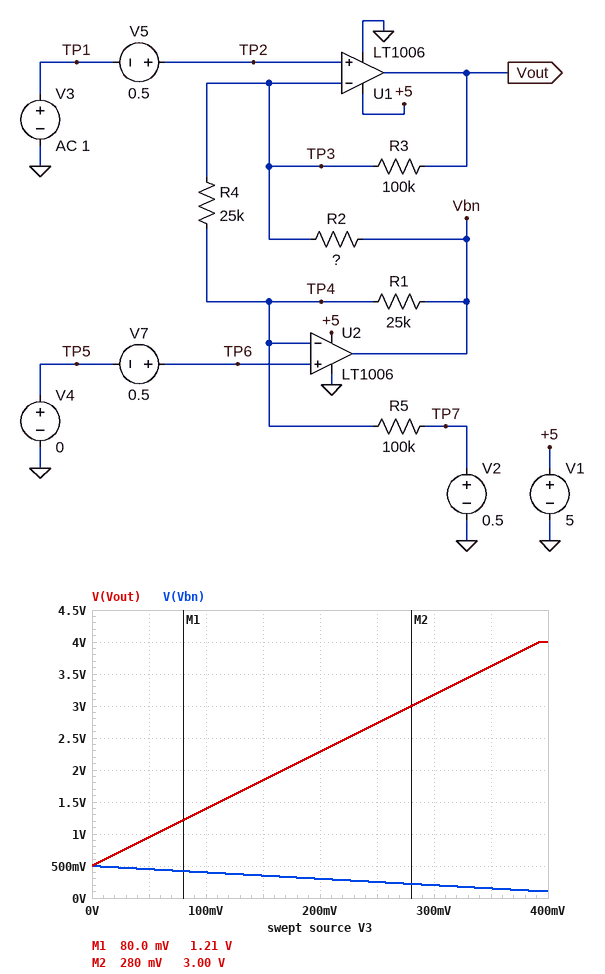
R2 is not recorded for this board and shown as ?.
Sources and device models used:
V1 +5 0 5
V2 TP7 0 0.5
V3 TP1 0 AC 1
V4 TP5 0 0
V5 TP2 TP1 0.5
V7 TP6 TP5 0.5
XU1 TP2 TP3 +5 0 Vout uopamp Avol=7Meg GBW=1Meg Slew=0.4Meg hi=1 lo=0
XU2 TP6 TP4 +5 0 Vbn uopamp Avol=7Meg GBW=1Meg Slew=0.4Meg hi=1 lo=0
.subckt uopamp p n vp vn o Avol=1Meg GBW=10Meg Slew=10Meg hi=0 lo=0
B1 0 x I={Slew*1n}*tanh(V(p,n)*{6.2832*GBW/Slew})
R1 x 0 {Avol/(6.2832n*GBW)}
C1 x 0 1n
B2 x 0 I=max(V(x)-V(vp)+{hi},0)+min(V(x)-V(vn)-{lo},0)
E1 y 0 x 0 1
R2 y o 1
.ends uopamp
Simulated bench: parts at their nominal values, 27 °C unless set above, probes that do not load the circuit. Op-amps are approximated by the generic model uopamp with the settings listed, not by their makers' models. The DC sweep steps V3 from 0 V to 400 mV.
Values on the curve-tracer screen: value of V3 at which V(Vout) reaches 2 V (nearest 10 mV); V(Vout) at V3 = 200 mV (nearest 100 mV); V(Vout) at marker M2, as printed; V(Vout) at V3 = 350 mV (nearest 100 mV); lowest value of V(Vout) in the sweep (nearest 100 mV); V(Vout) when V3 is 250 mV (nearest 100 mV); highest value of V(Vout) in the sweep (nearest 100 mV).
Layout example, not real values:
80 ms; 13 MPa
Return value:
170 mV; 2.3 V; 3.00 V; 3.6 V; 500 mV; 2.7 V; 4.0 V
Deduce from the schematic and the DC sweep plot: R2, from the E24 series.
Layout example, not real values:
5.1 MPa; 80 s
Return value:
51 kΩ
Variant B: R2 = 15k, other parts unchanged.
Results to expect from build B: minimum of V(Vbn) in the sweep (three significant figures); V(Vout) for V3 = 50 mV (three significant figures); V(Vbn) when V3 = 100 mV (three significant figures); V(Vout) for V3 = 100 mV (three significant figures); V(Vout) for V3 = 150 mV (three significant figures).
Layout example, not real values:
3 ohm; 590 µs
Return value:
309 mV; 1.42 V; 400 mV; 2.33 V; 3.25 V
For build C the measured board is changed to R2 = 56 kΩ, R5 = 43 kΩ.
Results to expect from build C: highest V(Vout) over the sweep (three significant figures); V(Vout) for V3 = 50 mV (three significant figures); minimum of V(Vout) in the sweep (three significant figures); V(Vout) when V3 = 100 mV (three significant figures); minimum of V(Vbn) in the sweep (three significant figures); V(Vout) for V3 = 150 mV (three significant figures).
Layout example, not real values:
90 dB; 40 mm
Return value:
3.93 V; 929 mV; 500 mV; 1.36 V; 100 mV; 1.79 V
